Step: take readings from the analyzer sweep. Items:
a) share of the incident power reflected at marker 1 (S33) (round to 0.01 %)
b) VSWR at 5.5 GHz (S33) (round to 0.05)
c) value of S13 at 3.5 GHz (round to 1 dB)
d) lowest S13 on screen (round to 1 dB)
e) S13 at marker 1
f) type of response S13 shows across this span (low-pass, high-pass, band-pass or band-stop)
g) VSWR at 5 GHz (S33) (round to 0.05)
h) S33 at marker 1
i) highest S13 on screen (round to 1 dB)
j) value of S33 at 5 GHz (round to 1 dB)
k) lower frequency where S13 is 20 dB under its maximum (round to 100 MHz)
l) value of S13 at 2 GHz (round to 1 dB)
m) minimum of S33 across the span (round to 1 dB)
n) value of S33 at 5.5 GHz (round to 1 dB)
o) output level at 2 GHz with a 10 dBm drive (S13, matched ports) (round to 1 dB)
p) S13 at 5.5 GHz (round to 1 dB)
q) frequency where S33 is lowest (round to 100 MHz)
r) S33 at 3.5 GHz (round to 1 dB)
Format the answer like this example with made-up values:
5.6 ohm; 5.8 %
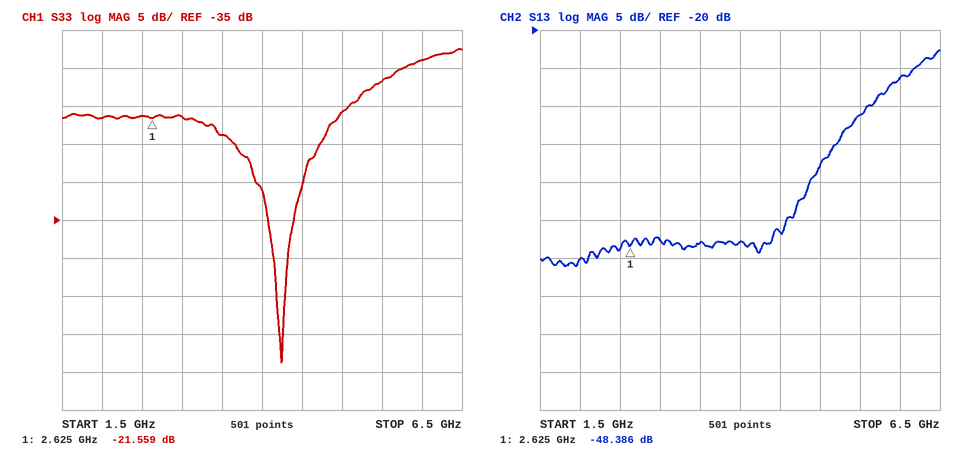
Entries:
0.70 %; 1.35; -48 dB; -51 dB; -48.386 dB; high-pass; 1.20; -21.559 dB; -23 dB; -21 dB; 4.7 GHz; -50 dB; -54 dB; -17 dB; -40 dBm; -31 dB; 4.2 GHz; -24 dB
